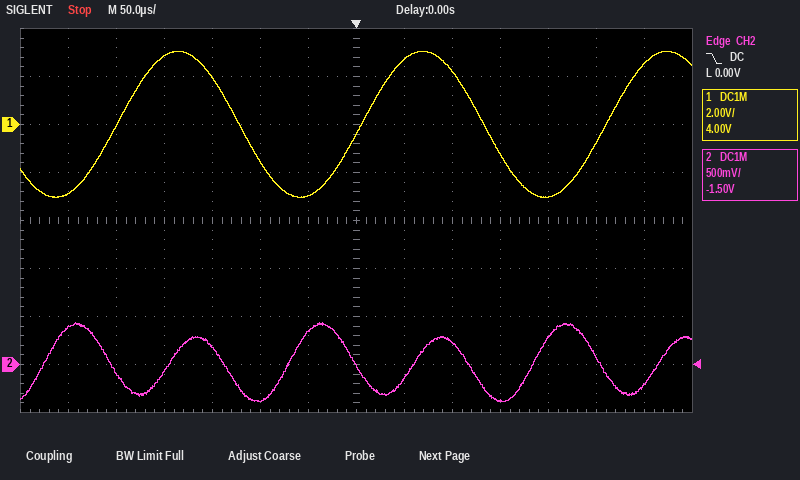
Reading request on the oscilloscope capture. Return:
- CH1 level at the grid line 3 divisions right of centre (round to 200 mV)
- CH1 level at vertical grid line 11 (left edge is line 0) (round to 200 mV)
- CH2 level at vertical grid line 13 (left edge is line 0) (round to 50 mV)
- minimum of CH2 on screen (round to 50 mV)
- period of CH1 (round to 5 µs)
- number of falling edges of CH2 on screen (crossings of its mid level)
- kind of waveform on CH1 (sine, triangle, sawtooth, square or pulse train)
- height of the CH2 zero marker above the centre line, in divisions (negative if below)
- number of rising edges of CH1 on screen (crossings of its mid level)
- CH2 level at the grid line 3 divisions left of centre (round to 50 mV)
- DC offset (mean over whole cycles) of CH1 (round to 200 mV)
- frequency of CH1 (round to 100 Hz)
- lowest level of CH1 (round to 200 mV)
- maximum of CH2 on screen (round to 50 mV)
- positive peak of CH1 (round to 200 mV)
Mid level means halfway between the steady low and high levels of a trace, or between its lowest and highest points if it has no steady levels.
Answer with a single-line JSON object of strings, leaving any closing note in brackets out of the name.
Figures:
{"CH1 level at the grid line 3 divisions right of centre": "-1.2 V", "CH1 level at vertical grid line 11 (left edge is line 0)": "-3.0 V", "CH2 level at vertical grid line 13 (left edge is line 0)": "-200 mV", "minimum of CH2 on screen": "-400 mV", "period of CH1": "255 µs", "number of falling edges of CH2 on screen": "5", "kind of waveform on CH1": "sine", "height of the CH2 zero marker above the centre line, in divisions": "-3.0 div", "number of rising edges of CH1 on screen": "3", "CH2 level at the grid line 3 divisions left of centre": "200 mV", "DC offset (mean over whole cycles) of CH1": "0.0 V", "frequency of CH1": "3.9 kHz", "lowest level of CH1": "-3.0 V", "maximum of CH2 on screen": "450 mV", "positive peak of CH1": "3.0 V"}
